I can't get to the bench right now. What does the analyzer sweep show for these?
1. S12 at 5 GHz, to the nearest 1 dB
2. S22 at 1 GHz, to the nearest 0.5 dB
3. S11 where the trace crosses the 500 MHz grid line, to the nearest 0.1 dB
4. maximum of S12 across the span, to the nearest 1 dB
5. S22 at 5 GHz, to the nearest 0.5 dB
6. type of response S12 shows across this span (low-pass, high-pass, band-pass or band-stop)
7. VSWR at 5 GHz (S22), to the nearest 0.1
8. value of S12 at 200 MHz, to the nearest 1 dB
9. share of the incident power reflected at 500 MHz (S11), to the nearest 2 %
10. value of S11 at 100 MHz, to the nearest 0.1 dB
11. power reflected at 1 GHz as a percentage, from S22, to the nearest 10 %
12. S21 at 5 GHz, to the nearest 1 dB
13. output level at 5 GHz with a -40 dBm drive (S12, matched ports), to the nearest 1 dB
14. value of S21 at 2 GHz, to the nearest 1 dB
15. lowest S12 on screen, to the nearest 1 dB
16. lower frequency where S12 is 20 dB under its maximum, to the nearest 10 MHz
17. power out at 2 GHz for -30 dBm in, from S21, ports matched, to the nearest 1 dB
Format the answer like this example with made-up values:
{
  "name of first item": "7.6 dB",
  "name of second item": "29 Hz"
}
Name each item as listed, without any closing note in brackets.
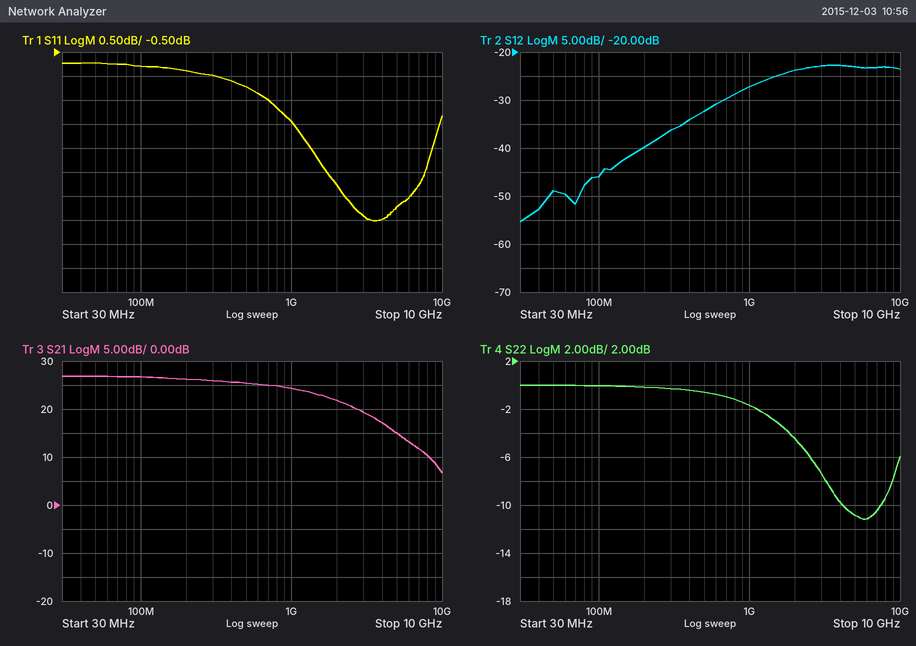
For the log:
{
  "S12 at 5 GHz, to the nearest 1 dB": "-23 dB",
  "S22 at 1 GHz, to the nearest 0.5 dB": "-1.5 dB",
  "S11 where the trace crosses the 500 MHz grid line, to the nearest 0.1 dB": "-1.2 dB",
  "maximum of S12 across the span, to the nearest 1 dB": "-23 dB",
  "S22 at 5 GHz, to the nearest 0.5 dB": "-11.0 dB",
  "type of response S12 shows across this span": "high-pass",
  "VSWR at 5 GHz (S22), to the nearest 0.1": "1.8",
  "value of S12 at 200 MHz, to the nearest 1 dB": "-40 dB",
  "share of the incident power reflected at 500 MHz (S11), to the nearest 2 %": "76 %",
  "value of S11 at 100 MHz, to the nearest 0.1 dB": "-0.8 dB",
  "power reflected at 1 GHz as a percentage, from S22, to the nearest 10 %": "70 %",
  "S21 at 5 GHz, to the nearest 1 dB": "15 dB",
  "output level at 5 GHz with a -40 dBm drive (S12, matched ports), to the nearest 1 dB": "-63 dBm",
  "value of S21 at 2 GHz, to the nearest 1 dB": "22 dB",
  "lowest S12 on screen, to the nearest 1 dB": "-55 dB",
  "lower frequency where S12 is 20 dB under its maximum, to the nearest 10 MHz": "140 MHz",
  "power out at 2 GHz for -30 dBm in, from S21, ports matched, to the nearest 1 dB": "-8 dBm"
}
